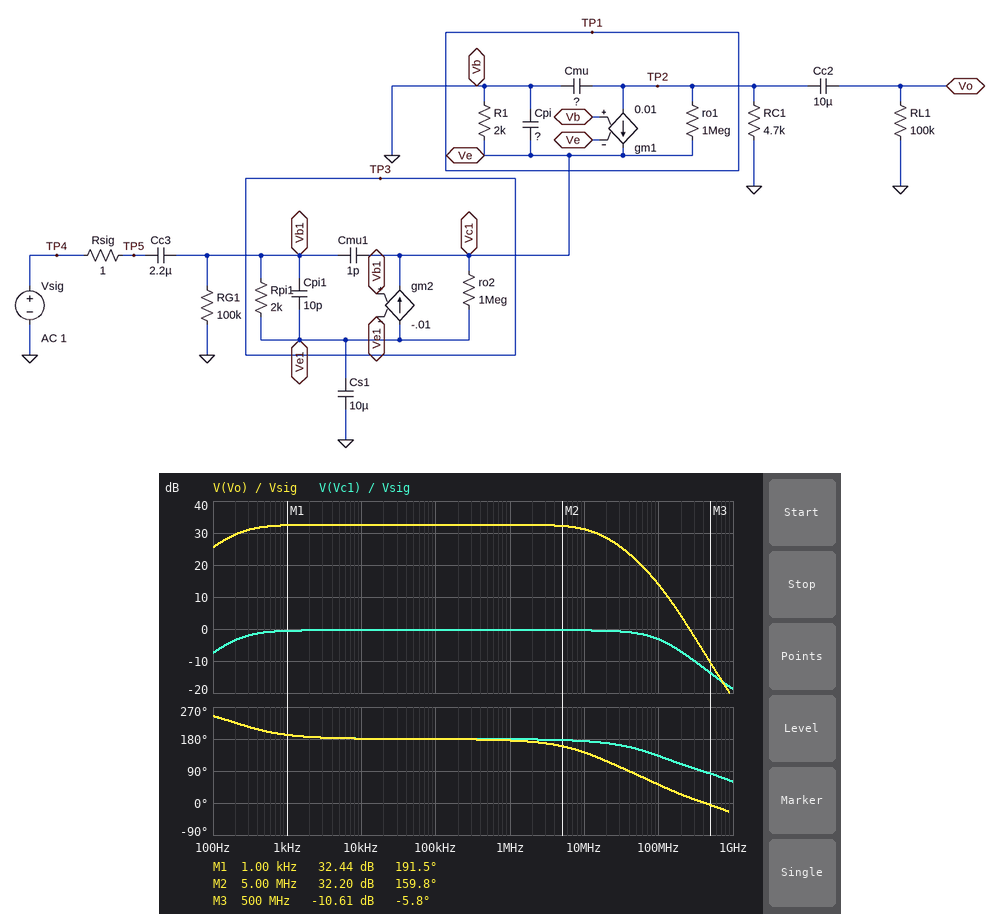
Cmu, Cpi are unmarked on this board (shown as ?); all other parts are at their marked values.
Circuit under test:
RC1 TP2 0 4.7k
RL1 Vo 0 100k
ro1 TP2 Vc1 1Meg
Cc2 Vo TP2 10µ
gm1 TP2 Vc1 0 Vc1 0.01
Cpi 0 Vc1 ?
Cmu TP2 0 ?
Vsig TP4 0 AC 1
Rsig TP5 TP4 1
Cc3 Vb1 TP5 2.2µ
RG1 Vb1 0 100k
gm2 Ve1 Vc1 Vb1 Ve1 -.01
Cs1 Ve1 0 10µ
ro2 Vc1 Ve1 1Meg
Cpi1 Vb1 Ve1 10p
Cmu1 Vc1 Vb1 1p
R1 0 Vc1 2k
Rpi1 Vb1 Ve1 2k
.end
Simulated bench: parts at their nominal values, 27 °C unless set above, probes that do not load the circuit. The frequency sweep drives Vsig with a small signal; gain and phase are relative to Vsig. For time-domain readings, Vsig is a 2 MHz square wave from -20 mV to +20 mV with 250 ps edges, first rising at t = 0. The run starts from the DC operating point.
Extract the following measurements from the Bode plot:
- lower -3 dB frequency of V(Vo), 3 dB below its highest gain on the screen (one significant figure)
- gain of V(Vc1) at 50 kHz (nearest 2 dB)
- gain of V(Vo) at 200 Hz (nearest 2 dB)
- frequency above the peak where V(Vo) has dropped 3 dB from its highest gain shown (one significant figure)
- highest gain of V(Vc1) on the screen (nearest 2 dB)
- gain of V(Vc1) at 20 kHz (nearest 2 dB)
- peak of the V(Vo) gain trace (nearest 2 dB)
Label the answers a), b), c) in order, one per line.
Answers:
a) 200 Hz
b) 0 dB
c) 30 dB
d) 20 MHz
e) 0 dB
f) 0 dB
g) 32 dB
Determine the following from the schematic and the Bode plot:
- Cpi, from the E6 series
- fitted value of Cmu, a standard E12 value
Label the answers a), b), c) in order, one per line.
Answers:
a) 15 pF
b) 2.2 pF
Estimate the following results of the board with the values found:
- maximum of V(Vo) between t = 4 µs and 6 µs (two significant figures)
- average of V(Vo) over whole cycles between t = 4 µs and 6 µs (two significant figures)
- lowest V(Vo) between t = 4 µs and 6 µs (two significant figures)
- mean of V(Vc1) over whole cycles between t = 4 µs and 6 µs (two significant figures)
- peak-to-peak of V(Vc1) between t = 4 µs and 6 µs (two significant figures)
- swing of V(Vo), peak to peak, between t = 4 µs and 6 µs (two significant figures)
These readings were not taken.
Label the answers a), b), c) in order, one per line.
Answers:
a) 6.8 mV
b) -850 mV
c) -1.7 V
d) -19 mV
e) 39 mV
f) 1.7 V
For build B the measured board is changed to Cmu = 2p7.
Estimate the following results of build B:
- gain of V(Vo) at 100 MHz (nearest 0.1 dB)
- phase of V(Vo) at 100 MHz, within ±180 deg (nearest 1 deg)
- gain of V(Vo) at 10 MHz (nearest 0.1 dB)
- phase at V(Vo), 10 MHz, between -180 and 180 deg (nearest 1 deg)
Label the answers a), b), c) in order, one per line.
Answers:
a) 12.1 dB
b) 50 deg
c) 30.6 dB
d) 137 deg
